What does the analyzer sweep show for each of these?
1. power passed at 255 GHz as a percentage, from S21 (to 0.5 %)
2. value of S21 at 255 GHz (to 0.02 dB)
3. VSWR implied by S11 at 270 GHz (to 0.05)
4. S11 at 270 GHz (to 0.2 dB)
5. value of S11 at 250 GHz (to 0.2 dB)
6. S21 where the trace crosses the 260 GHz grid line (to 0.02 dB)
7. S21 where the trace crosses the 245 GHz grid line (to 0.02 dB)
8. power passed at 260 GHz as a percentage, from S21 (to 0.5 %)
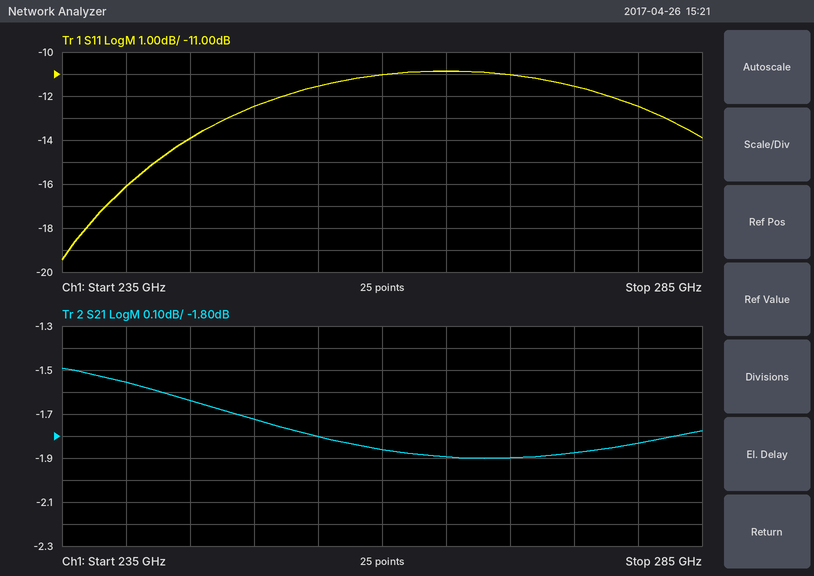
66.0 %
-1.80 dB
1.80
-11.0 dB
-12.4 dB
-1.86 dB
-1.64 dB
65.0 %
